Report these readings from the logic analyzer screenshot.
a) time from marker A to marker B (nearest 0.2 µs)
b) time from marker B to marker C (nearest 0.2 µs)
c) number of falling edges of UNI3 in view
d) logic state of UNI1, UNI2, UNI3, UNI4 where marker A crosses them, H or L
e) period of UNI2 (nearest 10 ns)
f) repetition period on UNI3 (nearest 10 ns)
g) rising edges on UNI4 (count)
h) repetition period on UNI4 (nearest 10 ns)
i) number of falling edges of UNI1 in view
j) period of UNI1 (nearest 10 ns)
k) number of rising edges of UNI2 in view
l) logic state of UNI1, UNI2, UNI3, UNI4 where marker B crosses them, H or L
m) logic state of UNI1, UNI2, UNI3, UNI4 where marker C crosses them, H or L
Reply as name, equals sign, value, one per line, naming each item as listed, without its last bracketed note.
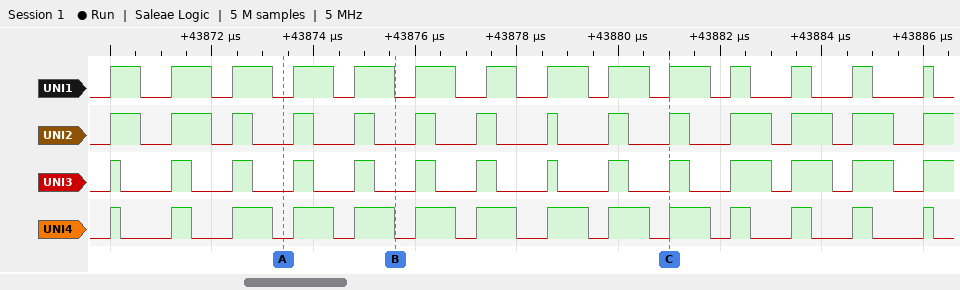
time from marker A to marker B = 2.2 µs
time from marker B to marker C = 5.4 µs
number of falling edges of UNI3 in view = 13
logic state of UNI1, UNI2, UNI3, UNI4 where marker A crosses them, H or L = UNI1=L, UNI2=L, UNI3=L, UNI4=L
period of UNI2 = 1230 ns
repetition period on UNI3 = 1230 ns
rising edges on UNI4 = 14
repetition period on UNI4 = 1230 ns
number of falling edges of UNI1 in view = 14
period of UNI1 = 1230 ns
number of rising edges of UNI2 in view = 14
logic state of UNI1, UNI2, UNI3, UNI4 where marker B crosses them, H or L = UNI1=L, UNI2=L, UNI3=L, UNI4=L
logic state of UNI1, UNI2, UNI3, UNI4 where marker C crosses them, H or L = UNI1=H, UNI2=H, UNI3=H, UNI4=H
